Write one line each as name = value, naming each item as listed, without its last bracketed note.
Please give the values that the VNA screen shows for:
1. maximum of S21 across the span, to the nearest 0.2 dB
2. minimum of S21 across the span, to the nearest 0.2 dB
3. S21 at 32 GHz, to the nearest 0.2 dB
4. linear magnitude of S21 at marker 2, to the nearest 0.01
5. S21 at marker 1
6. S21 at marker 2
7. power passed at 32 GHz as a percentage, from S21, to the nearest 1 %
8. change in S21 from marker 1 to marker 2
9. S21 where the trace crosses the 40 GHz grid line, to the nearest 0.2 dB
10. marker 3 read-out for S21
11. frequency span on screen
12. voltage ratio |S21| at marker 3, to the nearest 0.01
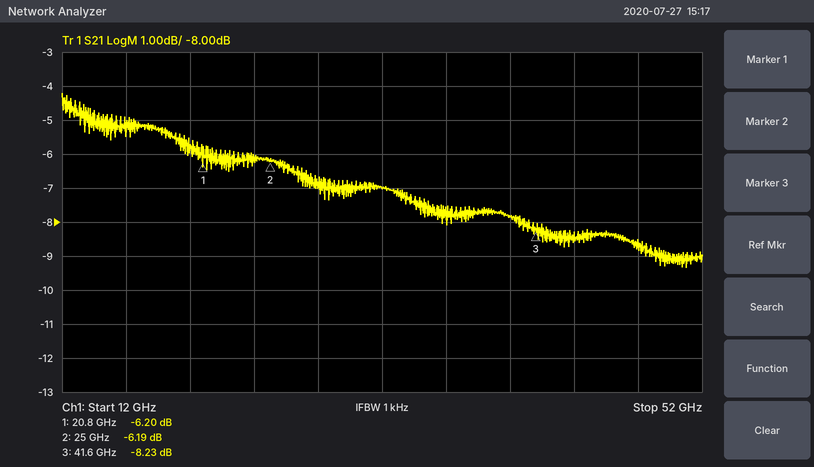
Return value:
maximum of S21 across the span, to the nearest 0.2 dB = -4.2 dB
minimum of S21 across the span, to the nearest 0.2 dB = -9.4 dB
S21 at 32 GHz, to the nearest 0.2 dB = -7.0 dB
linear magnitude of S21 at marker 2, to the nearest 0.01 = 0.49
S21 at marker 1 = -6.20 dB
S21 at marker 2 = -6.19 dB
power passed at 32 GHz as a percentage, from S21, to the nearest 1 % = 20 %
change in S21 from marker 1 to marker 2 = 0.01 dB
S21 where the trace crosses the 40 GHz grid line, to the nearest 0.2 dB = -7.8 dB
marker 3 read-out for S21 = -8.23 dB
frequency span on screen = 40 GHz
voltage ratio |S21| at marker 3, to the nearest 0.01 = 0.39
